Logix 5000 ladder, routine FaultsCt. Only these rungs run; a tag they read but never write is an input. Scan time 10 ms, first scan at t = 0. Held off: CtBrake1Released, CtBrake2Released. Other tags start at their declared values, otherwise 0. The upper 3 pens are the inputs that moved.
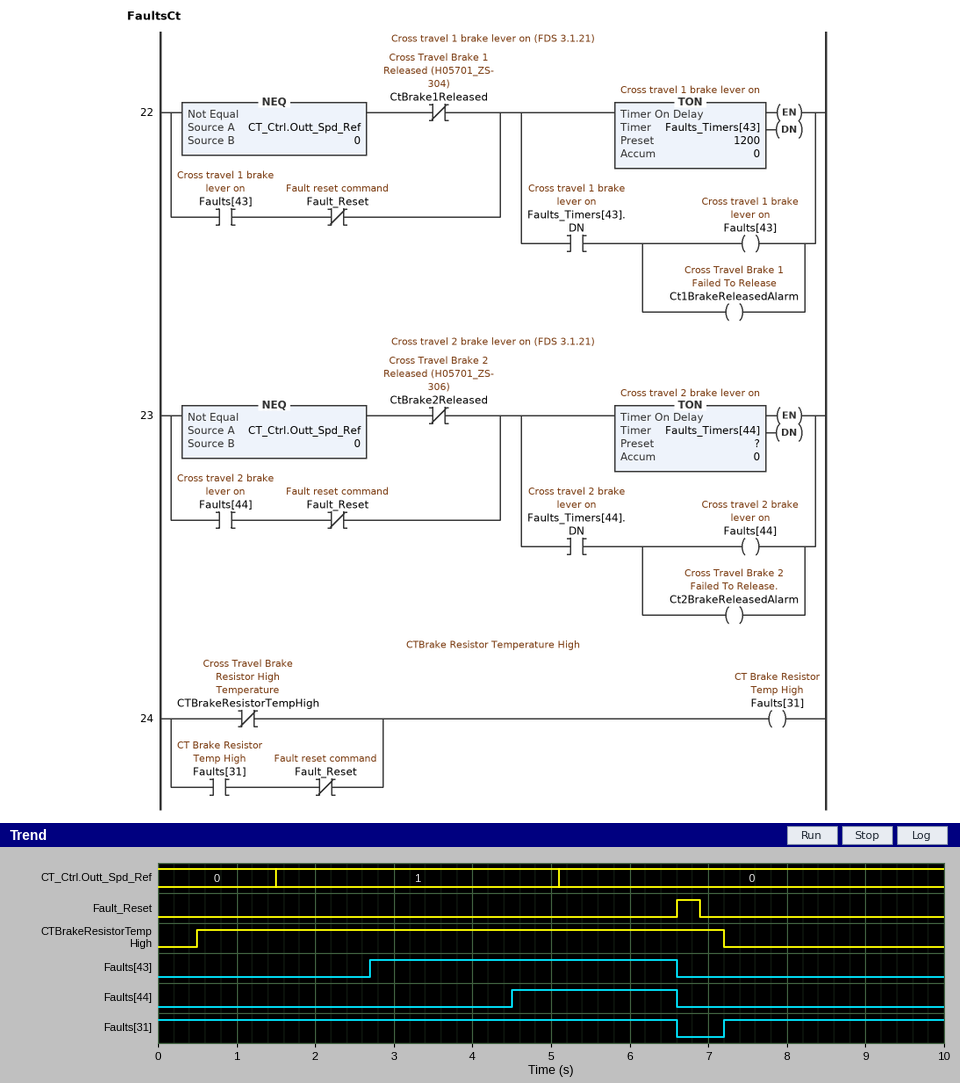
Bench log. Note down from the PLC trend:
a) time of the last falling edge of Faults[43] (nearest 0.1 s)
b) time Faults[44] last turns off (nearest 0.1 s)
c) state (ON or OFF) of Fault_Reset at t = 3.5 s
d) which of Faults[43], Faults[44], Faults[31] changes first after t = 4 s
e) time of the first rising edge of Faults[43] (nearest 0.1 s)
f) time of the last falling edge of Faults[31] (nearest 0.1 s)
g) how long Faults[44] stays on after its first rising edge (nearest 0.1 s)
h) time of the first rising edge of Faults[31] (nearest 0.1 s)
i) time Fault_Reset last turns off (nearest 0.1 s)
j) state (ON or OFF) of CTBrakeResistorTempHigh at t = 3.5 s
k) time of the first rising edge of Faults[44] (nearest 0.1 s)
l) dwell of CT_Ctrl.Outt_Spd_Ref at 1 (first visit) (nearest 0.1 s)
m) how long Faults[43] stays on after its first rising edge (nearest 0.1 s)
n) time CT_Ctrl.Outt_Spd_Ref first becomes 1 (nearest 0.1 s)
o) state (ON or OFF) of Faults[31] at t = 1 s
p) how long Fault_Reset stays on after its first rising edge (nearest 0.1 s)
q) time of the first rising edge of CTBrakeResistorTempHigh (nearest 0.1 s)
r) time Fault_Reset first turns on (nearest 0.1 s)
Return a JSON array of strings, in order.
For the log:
["6.6 s", "6.6 s", "OFF", "Faults[44]", "2.7 s", "6.6 s", "2.1 s", "7.2 s", "6.9 s", "ON", "4.5 s", "3.6 s", "3.9 s", "1.5 s", "ON", "0.3 s", "0.5 s", "6.6 s"]
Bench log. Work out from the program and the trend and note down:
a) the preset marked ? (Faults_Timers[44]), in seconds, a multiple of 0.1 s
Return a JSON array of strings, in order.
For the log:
["3.0 s"]
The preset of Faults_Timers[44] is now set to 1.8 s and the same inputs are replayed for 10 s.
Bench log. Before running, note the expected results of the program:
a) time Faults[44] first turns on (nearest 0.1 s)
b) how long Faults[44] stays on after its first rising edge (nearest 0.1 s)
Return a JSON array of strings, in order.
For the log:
["3.3 s", "3.3 s"]
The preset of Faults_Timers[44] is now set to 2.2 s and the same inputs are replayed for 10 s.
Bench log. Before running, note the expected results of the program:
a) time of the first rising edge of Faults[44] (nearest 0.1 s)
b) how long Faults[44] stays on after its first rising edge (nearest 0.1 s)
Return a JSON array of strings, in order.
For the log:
["3.7 s", "2.9 s"]
